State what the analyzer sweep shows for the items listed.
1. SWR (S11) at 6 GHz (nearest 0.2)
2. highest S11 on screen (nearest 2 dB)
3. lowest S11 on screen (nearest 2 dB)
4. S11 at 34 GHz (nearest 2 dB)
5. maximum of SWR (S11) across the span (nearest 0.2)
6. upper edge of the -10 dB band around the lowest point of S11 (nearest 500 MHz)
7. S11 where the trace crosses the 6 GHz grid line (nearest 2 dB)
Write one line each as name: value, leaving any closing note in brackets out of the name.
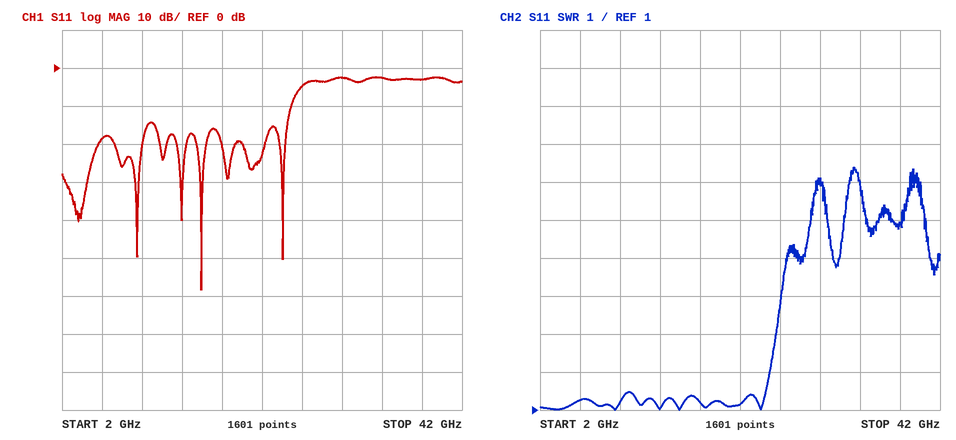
SWR (S11) at 6 GHz: 1.2
highest S11 on screen: -2 dB
lowest S11 on screen: -58 dB
S11 at 34 GHz: -2 dB
maximum of SWR (S11) across the span: 7.4
upper edge of the -10 dB band around the lowest point of S11: 25.0 GHz
S11 where the trace crosses the 6 GHz grid line: -18 dB
